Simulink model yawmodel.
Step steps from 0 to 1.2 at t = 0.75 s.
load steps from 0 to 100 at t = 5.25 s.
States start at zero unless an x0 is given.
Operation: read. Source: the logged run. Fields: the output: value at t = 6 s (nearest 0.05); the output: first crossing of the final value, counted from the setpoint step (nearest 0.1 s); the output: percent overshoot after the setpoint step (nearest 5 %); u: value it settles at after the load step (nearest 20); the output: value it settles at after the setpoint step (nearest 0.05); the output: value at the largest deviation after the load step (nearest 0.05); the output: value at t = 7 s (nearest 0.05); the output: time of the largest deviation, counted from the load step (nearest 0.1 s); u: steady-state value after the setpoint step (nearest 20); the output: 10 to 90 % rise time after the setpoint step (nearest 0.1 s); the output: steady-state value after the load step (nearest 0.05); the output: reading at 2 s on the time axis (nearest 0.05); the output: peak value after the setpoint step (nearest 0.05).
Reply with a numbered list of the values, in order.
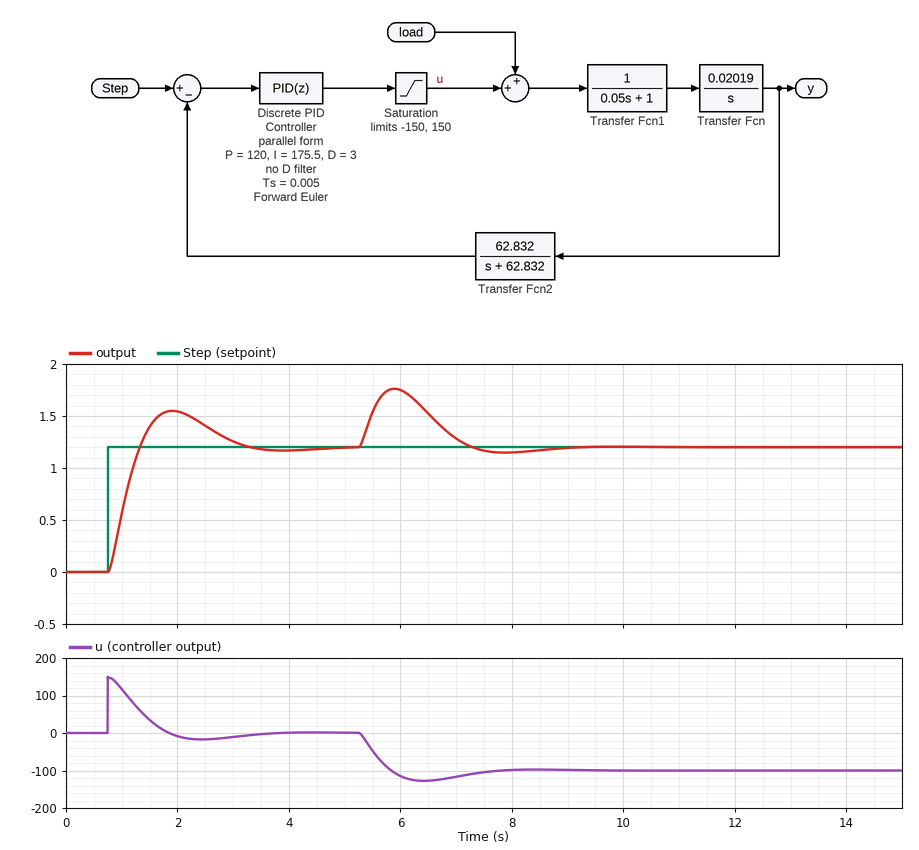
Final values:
1. 1.75
2. 0.6 s
3. 30 %
4. -100
5. 1.20
6. 1.75
7. 1.30
8. 0.6 s
9. 0
10. 0.4 s
11. 1.20
12. 1.55
13. 1.55
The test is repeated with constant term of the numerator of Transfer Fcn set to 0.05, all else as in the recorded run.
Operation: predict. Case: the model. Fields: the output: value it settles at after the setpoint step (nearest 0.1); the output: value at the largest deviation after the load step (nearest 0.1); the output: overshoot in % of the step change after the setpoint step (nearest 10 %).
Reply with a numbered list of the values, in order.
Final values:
1. 1.2
2. 1.9
3. 20 %
